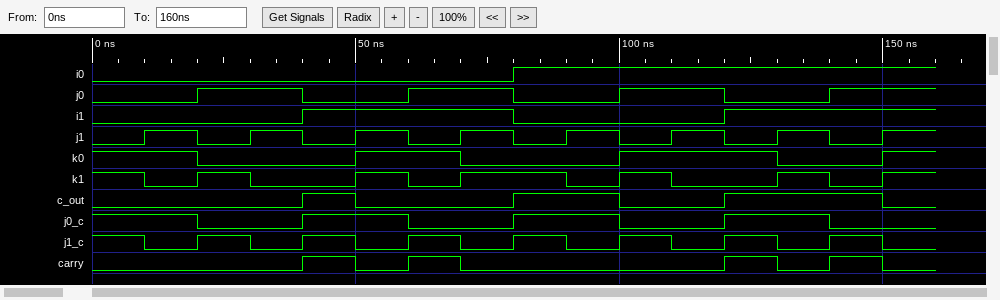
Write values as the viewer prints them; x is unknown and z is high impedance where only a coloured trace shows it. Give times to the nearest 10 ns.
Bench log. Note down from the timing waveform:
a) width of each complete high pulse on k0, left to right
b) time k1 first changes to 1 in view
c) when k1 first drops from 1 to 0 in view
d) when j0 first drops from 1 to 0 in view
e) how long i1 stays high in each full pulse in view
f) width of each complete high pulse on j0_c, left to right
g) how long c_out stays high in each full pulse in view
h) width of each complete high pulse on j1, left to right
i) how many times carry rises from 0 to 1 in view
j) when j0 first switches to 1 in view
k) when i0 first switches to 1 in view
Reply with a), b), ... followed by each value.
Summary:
a) 20 ns, 30 ns
b) 20 ns
c) 10 ns
d) 40 ns
e) 40 ns
f) 20 ns, 20 ns, 20 ns
g) 10 ns, 20 ns, 30 ns
h) 10 ns, 10 ns, 10 ns, 10 ns, 10 ns, 10 ns, 10 ns
i) 4
j) 20 ns
k) 80 ns
